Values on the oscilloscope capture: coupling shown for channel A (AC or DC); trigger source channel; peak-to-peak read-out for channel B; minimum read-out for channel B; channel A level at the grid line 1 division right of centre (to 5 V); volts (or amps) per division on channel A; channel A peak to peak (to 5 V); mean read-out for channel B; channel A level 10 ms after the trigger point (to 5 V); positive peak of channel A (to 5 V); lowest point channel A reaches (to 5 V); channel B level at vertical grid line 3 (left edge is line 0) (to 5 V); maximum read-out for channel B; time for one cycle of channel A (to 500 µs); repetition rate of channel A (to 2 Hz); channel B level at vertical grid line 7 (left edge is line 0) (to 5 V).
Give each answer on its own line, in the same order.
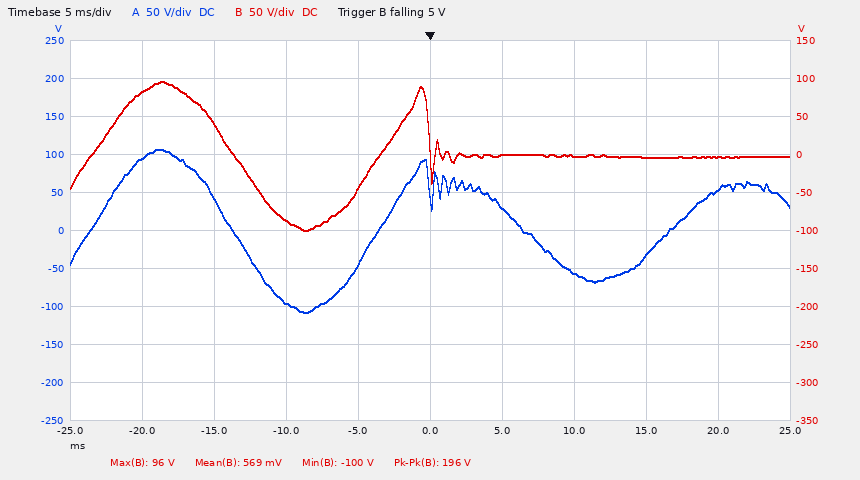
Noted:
DC
channel B
196 V
-100 V
30 V
50 V
215 V
569 mV
-55 V
105 V
-110 V
-85 V
96 V
20.0 ms
50 Hz
0 V
